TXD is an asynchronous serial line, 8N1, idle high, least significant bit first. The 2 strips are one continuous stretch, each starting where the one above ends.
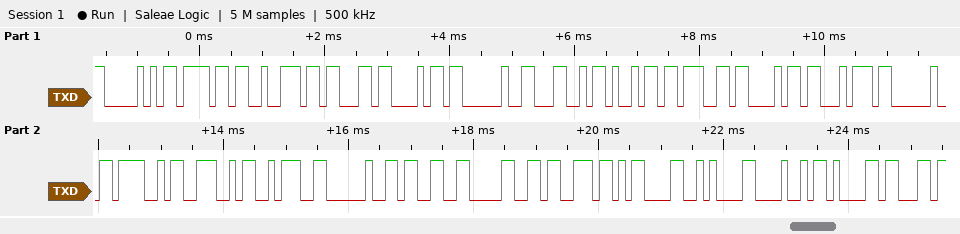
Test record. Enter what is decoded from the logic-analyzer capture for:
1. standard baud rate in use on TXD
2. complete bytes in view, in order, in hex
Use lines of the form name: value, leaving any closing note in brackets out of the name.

standard baud rate in use on TXD: 9600 baud
complete bytes in view, in order, in hex: 50 6F 72 63 68 20 4C 69 67 68 74 20 4F 4E 3A 20 33 30 73 0D 0A 48 61
